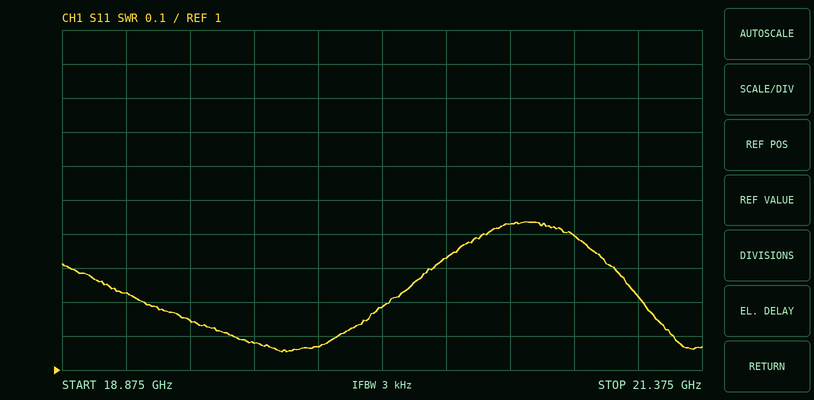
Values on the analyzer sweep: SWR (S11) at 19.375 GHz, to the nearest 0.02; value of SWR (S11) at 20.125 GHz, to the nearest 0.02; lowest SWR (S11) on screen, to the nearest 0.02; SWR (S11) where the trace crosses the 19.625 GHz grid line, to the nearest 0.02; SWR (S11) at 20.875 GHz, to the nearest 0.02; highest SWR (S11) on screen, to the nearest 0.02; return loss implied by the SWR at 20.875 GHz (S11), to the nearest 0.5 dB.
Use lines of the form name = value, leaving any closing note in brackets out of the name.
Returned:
SWR (S11) at 19.375 GHz, to the nearest 0.02 = 1.14
value of SWR (S11) at 20.125 GHz, to the nearest 0.02 = 1.18
lowest SWR (S11) on screen, to the nearest 0.02 = 1.06
SWR (S11) where the trace crosses the 19.625 GHz grid line, to the nearest 0.02 = 1.08
SWR (S11) at 20.875 GHz, to the nearest 0.02 = 1.40
highest SWR (S11) on screen, to the nearest 0.02 = 1.44
return loss implied by the SWR at 20.875 GHz (S11), to the nearest 0.5 dB = 15.5 dB
